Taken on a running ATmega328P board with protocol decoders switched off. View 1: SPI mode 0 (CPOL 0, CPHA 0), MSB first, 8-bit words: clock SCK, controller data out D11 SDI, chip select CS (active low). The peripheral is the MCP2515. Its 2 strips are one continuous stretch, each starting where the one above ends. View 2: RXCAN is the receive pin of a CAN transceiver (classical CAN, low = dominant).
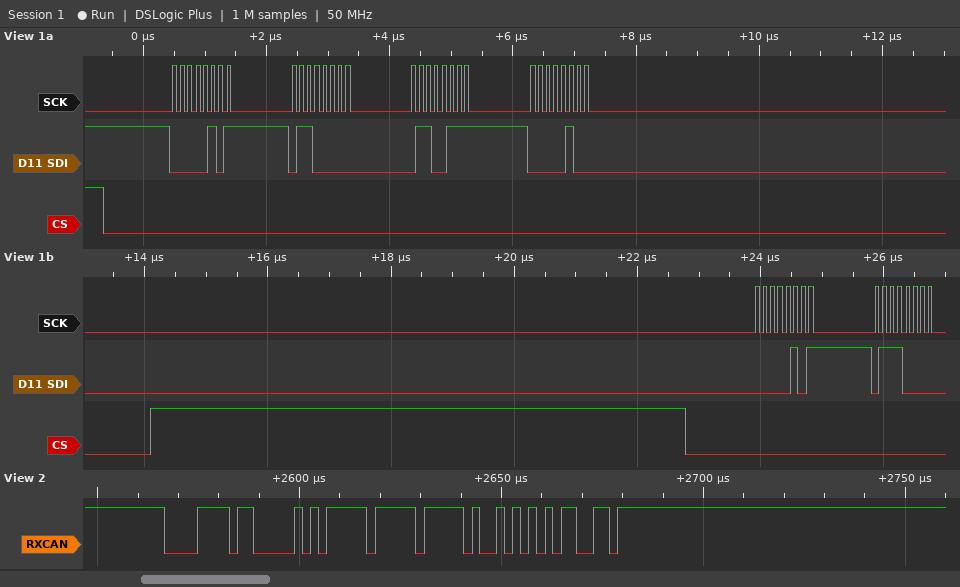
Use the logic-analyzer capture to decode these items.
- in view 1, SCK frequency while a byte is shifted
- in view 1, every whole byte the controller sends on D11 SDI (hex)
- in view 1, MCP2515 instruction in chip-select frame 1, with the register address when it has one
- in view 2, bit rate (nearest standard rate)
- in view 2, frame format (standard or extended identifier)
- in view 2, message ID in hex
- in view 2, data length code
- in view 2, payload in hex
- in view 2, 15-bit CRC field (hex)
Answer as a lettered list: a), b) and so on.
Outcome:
a) 8 MHz
b) 05 60 67 04 05 70
c) BIT MODIFY 0x60
d) 500 kbit/s
e) standard
f) 0x0F6
g) 2
h) FF FF
i) 0x1559
